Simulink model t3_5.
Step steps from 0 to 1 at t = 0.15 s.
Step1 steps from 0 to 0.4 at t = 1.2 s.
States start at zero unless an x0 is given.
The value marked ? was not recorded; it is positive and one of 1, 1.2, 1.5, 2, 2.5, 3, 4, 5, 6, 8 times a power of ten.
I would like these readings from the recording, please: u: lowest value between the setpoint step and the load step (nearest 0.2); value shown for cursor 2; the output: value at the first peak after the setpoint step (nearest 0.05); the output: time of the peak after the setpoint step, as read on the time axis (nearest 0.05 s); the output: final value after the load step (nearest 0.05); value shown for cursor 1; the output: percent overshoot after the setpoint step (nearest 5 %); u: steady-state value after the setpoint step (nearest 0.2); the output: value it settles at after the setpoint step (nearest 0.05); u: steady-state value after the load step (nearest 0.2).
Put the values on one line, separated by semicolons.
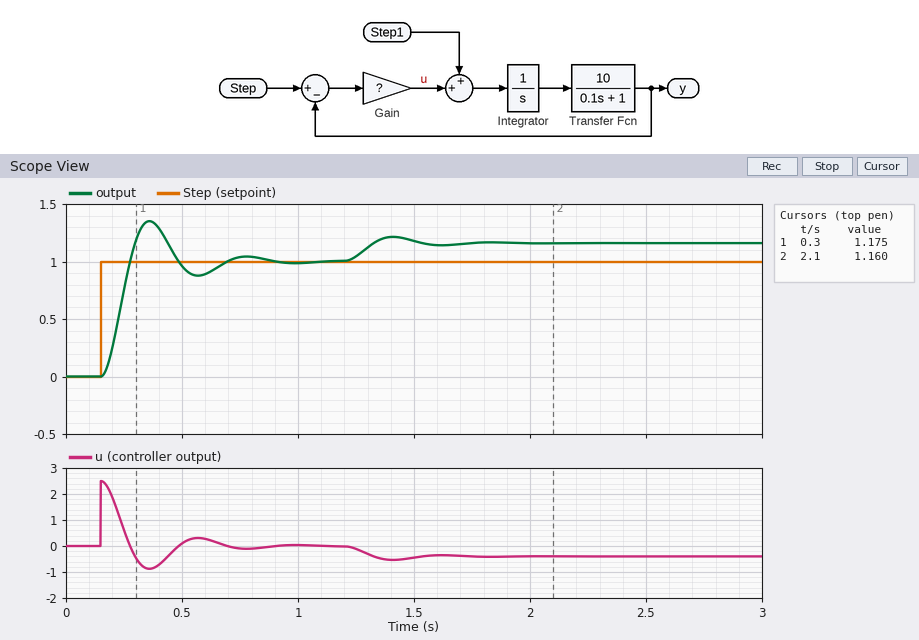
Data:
-0.8; 1.160; 1.35; 0.35 s; 1.15; 1.175; 35 %; 0.0; 1.00; -0.4
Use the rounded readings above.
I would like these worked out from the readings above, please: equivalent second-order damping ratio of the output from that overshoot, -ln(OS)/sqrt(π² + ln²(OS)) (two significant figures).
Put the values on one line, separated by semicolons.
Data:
0.32
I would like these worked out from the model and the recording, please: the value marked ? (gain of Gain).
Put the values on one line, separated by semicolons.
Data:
2.5
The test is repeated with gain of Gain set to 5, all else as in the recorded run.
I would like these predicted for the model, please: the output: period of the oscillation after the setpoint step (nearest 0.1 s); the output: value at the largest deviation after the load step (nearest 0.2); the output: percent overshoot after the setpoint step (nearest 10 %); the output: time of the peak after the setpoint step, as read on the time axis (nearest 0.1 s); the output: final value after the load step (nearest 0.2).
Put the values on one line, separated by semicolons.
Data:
0.3 s; 1.2; 50 %; 0.3 s; 1.0
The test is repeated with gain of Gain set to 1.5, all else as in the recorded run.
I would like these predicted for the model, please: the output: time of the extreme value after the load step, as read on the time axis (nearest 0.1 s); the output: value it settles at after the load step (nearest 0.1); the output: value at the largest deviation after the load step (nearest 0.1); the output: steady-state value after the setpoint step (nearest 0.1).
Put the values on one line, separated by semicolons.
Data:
1.5 s; 1.3; 1.3; 1.0
